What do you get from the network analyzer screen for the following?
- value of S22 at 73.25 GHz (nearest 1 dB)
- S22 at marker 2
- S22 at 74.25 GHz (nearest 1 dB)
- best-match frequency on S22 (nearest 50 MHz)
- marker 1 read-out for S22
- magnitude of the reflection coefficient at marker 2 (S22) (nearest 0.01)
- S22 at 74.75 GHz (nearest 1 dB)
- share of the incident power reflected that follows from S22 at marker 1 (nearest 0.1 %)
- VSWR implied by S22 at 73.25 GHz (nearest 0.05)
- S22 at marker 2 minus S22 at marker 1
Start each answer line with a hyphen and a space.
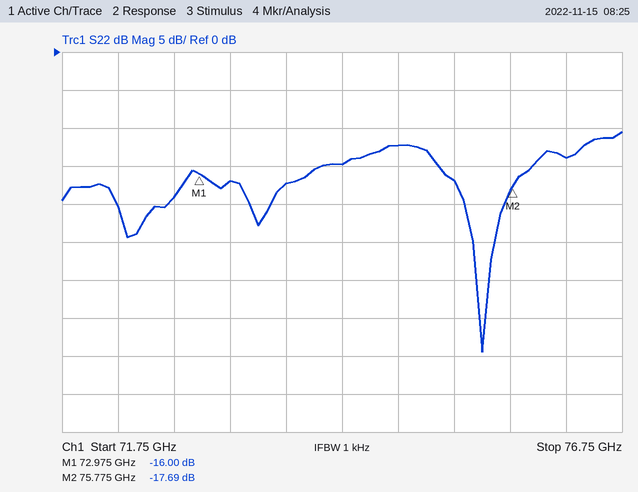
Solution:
- -17 dB
- -17.69 dB
- -15 dB
- 75.50 GHz
- -16.00 dB
- 0.13
- -12 dB
- 2.5 %
- 1.35
- -1.69 dB
